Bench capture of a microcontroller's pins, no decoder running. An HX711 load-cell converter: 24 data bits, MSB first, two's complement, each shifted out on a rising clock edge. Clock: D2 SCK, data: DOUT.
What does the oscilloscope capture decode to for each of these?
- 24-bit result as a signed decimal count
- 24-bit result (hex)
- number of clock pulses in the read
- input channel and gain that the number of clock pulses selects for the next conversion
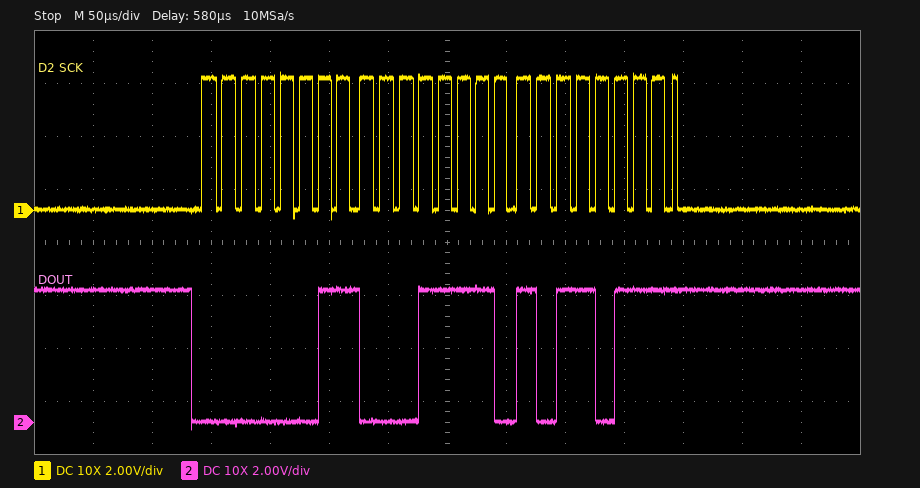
204471
0x031EB7
25
channel A, gain 128
